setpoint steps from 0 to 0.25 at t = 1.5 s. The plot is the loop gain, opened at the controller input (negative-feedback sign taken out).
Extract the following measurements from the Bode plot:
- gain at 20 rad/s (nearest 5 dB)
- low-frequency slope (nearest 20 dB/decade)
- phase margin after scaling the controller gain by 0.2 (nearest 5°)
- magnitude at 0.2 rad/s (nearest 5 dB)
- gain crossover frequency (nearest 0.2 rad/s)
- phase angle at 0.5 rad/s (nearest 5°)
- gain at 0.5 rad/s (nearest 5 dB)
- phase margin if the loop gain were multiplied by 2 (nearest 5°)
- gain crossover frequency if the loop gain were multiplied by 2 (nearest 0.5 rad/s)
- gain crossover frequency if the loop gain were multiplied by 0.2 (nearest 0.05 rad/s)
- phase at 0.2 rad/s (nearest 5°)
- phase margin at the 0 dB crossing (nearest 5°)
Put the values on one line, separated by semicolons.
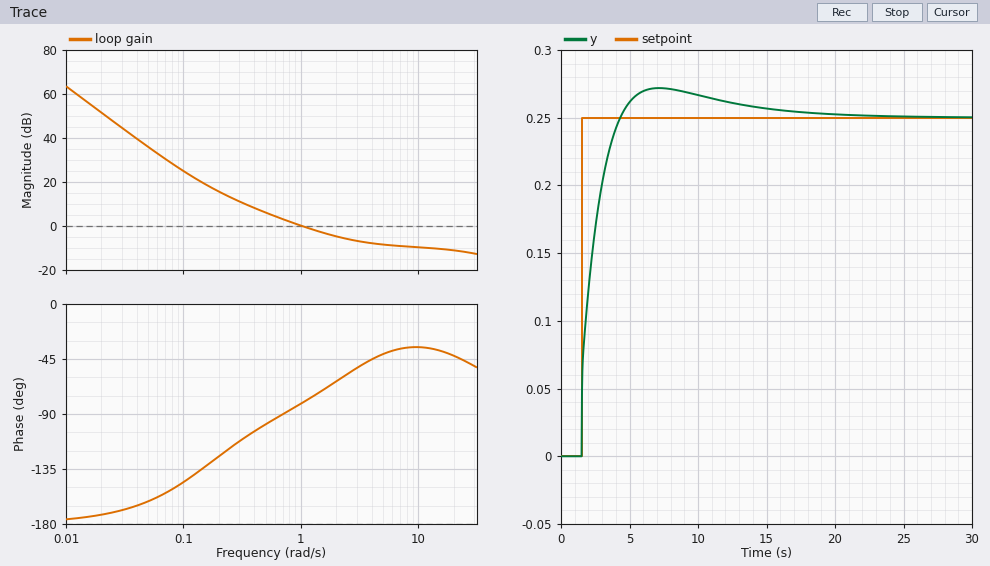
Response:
-10 dB; -40 dB/decade; 60°; 15 dB; 1.0 rad/s; -100°; 5 dB; 125°; 2.5 rad/s; 0.25 rad/s; -125°; 100°
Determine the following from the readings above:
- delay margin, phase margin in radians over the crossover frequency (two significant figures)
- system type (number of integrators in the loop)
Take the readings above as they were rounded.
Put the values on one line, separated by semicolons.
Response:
1.7 s; 2
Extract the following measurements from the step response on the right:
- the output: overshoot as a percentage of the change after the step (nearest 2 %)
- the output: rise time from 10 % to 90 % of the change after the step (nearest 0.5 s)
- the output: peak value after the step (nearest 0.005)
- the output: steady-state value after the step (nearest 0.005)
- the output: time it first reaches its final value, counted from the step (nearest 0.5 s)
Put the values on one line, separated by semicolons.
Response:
8 %; 2.0 s; 0.270; 0.250; 3.0 s
